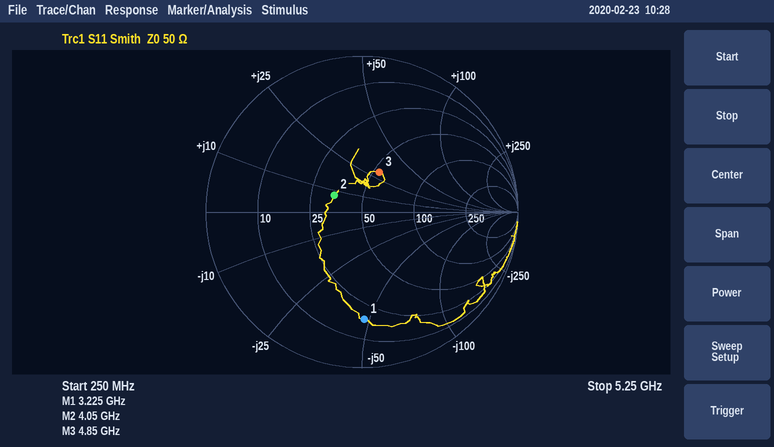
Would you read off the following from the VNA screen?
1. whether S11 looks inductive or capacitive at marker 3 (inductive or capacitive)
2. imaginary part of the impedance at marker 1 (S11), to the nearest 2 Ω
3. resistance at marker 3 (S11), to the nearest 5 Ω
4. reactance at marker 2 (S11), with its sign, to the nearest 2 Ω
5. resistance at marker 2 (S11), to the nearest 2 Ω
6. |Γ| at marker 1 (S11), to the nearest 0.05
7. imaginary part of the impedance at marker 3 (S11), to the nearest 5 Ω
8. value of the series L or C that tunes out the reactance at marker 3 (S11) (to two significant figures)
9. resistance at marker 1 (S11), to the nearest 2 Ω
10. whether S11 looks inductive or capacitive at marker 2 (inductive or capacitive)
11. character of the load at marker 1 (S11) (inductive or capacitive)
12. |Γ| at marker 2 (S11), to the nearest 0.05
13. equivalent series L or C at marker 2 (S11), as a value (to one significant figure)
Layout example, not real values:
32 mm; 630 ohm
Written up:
inductive; -48 Ω; 55 Ω; +8 Ω; 34 Ω; 0.70; +30 Ω; 1.1 pF; 18 Ω; inductive; capacitive; 0.20; 300 pH
